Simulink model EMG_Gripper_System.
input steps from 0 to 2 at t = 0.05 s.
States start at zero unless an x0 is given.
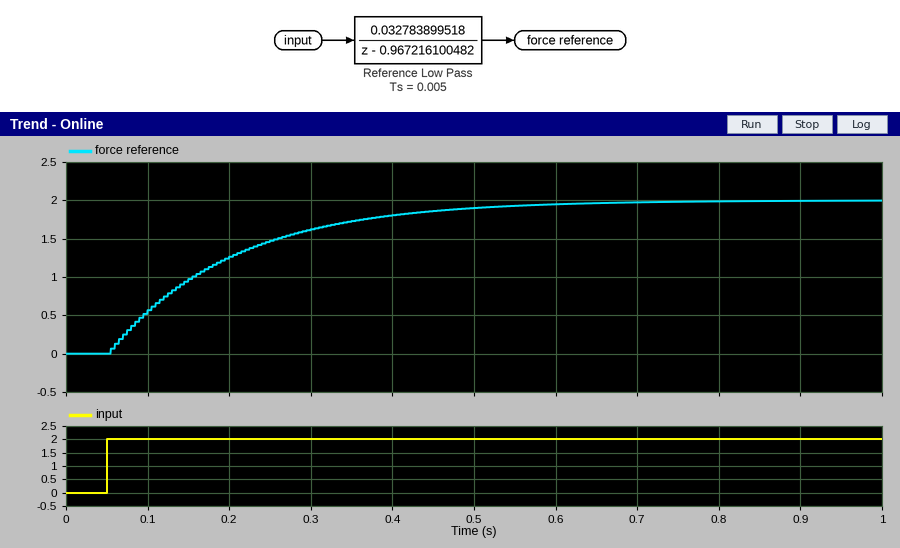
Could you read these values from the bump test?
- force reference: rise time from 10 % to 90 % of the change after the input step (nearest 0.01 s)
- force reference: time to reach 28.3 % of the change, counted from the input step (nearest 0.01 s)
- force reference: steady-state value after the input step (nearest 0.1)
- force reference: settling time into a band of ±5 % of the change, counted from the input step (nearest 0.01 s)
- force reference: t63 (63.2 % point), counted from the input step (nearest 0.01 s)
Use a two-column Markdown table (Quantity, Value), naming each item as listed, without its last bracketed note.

| Quantity | Value |
|---|---|
| force reference: rise time from 10 % to 90 % of the change after the input step | 0.33 s |
| force reference: time to reach 28.3 % of the change, counted from the input step | 0.05 s |
| force reference: steady-state value after the input step | 2.0 |
| force reference: settling time into a band of ±5 % of the change, counted from the input step | 0.45 s |
| force reference: t63 (63.2 % point), counted from the input step | 0.15 s |
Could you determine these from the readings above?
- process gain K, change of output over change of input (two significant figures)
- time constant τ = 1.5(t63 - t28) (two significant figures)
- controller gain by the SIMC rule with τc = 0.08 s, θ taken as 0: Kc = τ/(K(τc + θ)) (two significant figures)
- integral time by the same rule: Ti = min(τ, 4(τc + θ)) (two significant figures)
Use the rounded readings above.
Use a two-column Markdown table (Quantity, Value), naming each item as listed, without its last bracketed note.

| Quantity | Value |
|---|---|
| process gain K, change of output over change of input | 1.0 |
| time constant τ = 1.5(t63 - t28) | 0.15 s |
| controller gain by the SIMC rule with τc = 0.08 s, θ taken as 0: Kc = τ/(K(τc + θ)) | 1.9 |
| integral time by the same rule: Ti = min(τ, 4(τc + θ)) | 0.15 s |
